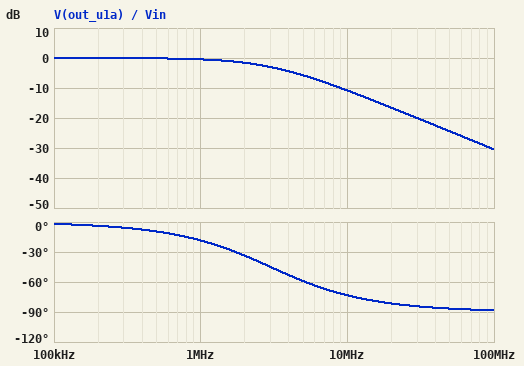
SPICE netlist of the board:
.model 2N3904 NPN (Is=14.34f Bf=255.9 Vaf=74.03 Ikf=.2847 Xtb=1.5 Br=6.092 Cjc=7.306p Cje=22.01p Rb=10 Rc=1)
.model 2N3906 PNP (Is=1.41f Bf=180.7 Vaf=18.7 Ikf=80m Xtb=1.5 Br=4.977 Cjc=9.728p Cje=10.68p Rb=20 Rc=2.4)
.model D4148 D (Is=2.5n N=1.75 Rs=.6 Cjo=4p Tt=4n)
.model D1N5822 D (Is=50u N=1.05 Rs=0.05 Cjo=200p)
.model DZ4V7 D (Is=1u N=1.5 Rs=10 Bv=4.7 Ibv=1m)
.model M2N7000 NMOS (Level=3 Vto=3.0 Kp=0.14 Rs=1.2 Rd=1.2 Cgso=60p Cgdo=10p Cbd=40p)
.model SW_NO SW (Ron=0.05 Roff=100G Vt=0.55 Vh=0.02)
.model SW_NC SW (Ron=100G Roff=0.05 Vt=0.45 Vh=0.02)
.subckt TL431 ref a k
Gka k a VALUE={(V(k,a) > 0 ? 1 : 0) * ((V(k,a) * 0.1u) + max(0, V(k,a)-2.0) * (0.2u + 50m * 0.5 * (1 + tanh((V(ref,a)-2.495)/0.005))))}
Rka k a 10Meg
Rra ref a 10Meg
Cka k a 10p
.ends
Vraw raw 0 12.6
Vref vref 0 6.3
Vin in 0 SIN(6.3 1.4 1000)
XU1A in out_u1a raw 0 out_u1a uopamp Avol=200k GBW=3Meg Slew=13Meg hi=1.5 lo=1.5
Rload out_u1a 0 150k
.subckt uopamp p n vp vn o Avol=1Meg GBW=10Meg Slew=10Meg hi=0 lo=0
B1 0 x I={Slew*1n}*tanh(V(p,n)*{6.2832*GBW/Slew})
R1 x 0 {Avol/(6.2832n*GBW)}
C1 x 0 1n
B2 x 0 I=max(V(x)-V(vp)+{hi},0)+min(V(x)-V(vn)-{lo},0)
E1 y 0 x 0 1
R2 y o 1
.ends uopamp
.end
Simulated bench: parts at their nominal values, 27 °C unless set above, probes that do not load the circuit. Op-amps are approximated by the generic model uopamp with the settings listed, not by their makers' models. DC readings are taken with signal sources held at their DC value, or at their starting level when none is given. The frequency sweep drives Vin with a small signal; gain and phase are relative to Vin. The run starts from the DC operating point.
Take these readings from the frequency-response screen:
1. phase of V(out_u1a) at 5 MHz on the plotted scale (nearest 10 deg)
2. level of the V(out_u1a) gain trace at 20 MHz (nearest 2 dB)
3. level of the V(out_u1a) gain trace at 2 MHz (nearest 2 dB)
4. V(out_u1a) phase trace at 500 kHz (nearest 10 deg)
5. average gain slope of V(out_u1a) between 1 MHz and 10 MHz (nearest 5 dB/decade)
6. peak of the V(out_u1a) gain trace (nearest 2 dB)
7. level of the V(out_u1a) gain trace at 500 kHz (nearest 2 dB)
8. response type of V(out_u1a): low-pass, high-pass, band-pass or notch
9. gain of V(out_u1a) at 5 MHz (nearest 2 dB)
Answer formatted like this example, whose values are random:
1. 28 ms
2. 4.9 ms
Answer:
1. -60 deg
2. -16 dB
3. -2 dB
4. -10 deg
5. -10 dB/decade
6. 0 dB
7. 0 dB
8. low-pass
9. -6 dB
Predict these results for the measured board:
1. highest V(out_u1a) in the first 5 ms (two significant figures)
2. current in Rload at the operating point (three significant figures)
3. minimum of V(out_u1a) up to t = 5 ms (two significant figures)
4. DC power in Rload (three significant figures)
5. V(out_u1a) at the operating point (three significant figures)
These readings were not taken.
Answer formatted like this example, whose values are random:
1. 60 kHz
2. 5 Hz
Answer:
1. 7.7 V
2. 42.0 µA
3. 4.9 V
4. 265 µW
5. 6.30 V
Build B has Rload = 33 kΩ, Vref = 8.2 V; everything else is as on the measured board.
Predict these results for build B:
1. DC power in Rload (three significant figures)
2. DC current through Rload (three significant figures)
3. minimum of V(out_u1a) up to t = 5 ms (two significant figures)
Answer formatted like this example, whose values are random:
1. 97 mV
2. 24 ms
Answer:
1. 1.20 mW
2. 191 µA
3. 4.9 V
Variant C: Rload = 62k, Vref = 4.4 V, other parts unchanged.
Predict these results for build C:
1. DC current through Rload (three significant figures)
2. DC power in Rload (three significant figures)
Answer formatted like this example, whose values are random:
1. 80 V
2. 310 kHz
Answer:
1. 102 µA
2. 640 µW
